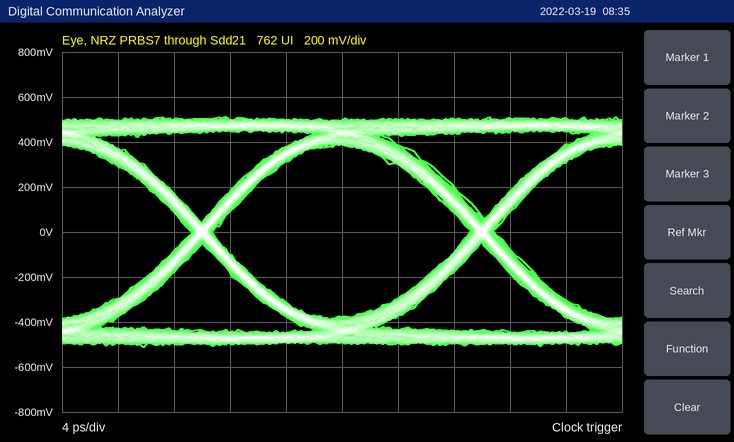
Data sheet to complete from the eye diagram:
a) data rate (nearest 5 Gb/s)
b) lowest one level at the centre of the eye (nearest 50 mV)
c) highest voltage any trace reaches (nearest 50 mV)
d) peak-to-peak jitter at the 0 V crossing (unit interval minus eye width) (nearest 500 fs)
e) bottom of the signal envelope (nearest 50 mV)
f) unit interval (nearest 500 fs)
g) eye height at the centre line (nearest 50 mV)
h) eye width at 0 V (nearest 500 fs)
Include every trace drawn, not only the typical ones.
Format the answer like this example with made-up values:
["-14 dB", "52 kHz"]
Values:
["50 Gb/s", "400 mV", "500 mV", "1.5 ps", "-500 mV", "20.0 ps", "750 mV", "18.5 ps"]
